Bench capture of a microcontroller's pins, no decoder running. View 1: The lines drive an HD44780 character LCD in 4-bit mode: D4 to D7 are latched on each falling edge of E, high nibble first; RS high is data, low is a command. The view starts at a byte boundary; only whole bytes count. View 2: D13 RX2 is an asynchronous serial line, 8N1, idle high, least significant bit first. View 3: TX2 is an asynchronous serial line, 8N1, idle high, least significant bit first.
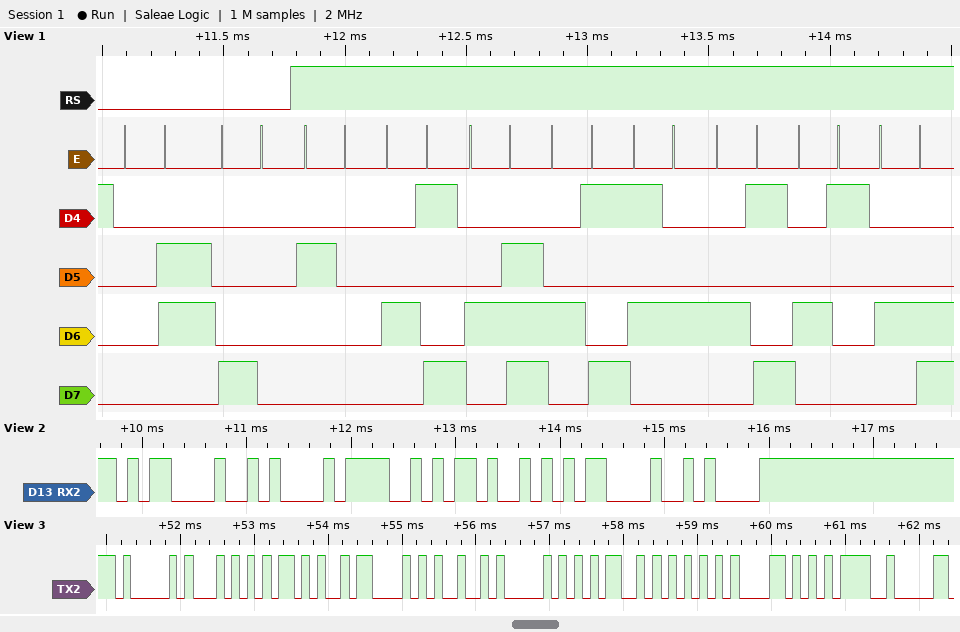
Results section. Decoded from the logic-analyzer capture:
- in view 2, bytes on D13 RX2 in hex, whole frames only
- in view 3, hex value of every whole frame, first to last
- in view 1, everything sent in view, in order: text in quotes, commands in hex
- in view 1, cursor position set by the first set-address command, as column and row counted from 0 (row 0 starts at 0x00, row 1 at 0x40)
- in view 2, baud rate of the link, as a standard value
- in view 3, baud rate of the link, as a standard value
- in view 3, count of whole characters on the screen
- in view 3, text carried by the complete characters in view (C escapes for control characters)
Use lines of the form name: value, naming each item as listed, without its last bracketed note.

in view 2, bytes on D13 RX2 in hex, whole frames only: 0x0D 0x0A 0x4F 0x4B 0x0D 0x0A
in view 3, hex value of every whole frame, first to last: 41 54 2B 43 49 50 4D 55 58 3D
in view 1, everything sent in view, in order: text in quotes, commands in hex: 0x06 0x80 " INITIAL"
in view 1, cursor position set by the first set-address command, as column and row counted from 0: column 0, row 0
in view 2, baud rate of the link, as a standard value: 9600 baud
in view 3, baud rate of the link, as a standard value: 9600 baud
in view 3, count of whole characters on the screen: 10
in view 3, text carried by the complete characters in view: "AT+CIPMUX="
